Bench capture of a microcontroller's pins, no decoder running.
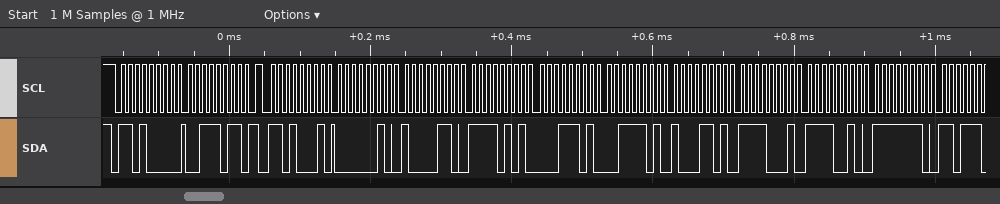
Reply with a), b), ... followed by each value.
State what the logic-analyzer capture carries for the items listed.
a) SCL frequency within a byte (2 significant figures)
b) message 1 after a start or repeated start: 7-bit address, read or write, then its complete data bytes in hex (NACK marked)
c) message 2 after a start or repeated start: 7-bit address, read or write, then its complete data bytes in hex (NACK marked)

a) 100 kHz
b) 0x68 write: 3B
c) 0x68 read: 02 86 F5 1D 3D 8D F1 F2 FE
